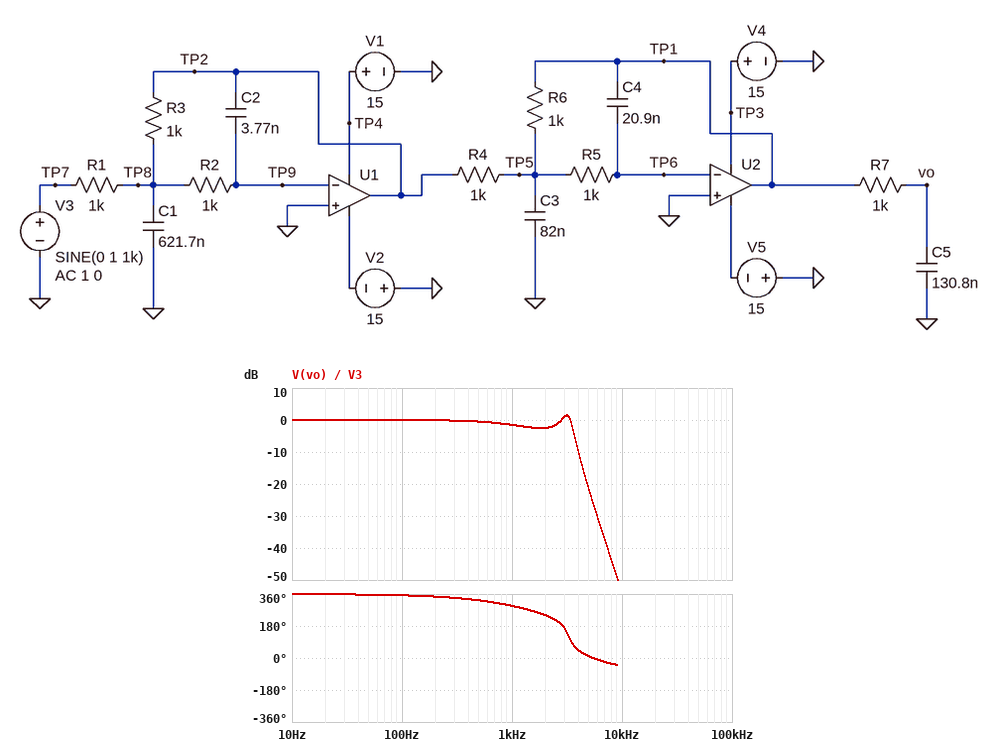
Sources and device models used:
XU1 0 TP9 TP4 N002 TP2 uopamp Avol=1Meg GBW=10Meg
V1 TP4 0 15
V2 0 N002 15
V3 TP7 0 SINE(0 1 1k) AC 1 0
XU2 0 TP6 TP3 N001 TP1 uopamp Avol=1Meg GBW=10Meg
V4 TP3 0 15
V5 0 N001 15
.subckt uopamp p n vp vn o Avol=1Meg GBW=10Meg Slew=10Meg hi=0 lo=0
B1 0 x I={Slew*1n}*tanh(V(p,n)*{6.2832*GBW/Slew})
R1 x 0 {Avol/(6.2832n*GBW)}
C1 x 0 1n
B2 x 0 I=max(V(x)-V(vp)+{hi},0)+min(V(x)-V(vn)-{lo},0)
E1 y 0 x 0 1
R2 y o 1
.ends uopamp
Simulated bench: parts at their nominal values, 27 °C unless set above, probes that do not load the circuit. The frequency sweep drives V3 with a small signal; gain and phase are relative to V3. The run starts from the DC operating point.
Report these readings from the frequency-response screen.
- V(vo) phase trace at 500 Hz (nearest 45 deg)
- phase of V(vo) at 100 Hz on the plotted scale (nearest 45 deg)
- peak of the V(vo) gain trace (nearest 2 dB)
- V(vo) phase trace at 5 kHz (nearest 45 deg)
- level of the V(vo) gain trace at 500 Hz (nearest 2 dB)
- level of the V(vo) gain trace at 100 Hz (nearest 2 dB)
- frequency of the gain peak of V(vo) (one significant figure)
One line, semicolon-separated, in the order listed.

315 deg; 360 deg; 2 dB; 0 deg; 0 dB; 0 dB; 3 kHz
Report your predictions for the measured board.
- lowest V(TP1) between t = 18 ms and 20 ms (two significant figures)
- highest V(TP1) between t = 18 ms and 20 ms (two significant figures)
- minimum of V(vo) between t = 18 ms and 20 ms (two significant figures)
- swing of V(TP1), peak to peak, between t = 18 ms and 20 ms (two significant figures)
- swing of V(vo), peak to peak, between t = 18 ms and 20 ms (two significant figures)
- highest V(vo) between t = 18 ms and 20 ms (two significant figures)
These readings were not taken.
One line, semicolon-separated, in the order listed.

-1.1 V; 1.1 V; -840 mV; 2.2 V; 1.7 V; 840 mV
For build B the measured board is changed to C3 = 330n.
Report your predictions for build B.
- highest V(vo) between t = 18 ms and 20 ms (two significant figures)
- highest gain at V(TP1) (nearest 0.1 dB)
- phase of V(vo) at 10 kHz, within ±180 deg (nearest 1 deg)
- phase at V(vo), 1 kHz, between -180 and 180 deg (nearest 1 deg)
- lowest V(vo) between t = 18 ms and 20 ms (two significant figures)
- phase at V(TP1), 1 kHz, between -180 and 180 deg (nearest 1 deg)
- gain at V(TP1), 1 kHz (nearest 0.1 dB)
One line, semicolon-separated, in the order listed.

1.0 V; 6.1 dB; -70 deg; -72 deg; -1.0 V; -33 deg; 2.5 dB
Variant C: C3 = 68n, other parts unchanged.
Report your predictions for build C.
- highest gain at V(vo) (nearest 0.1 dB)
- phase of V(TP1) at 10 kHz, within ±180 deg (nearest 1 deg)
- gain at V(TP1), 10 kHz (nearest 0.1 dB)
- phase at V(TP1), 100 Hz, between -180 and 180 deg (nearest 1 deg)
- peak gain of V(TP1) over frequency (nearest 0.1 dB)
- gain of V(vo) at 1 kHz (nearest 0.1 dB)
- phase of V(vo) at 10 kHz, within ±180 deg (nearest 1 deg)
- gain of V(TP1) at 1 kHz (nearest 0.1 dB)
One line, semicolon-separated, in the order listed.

1.2 dB; 45 deg; -34.1 dB; -3 deg; 10.2 dB; -1.6 dB; -38 deg; 0.6 dB
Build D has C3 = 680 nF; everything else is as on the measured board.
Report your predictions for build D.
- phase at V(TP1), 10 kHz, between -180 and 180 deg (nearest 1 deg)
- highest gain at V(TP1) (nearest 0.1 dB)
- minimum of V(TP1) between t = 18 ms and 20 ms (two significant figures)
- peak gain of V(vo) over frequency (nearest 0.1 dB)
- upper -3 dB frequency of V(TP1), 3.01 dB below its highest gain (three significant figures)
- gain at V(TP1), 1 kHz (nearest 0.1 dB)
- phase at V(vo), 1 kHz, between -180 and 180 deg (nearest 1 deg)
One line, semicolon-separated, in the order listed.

9 deg; 7.2 dB; -1.9 V; 4.1 dB; 1.63 kHz; 5.4 dB; -86 deg
